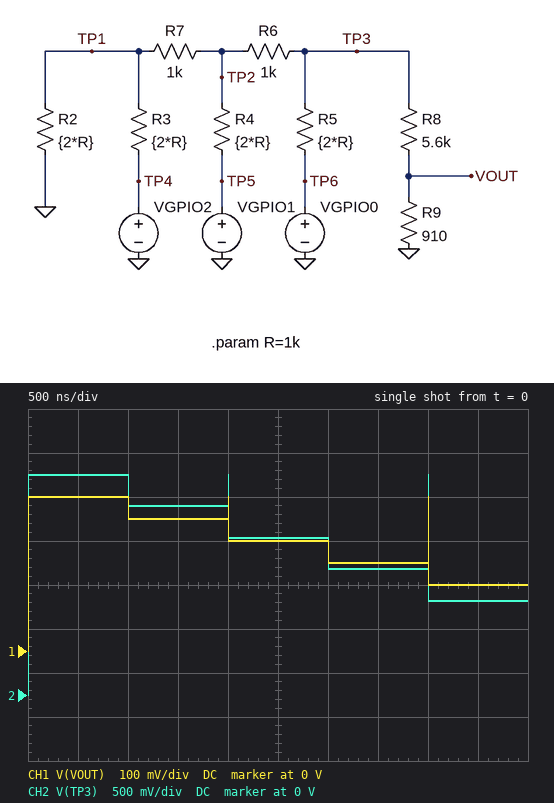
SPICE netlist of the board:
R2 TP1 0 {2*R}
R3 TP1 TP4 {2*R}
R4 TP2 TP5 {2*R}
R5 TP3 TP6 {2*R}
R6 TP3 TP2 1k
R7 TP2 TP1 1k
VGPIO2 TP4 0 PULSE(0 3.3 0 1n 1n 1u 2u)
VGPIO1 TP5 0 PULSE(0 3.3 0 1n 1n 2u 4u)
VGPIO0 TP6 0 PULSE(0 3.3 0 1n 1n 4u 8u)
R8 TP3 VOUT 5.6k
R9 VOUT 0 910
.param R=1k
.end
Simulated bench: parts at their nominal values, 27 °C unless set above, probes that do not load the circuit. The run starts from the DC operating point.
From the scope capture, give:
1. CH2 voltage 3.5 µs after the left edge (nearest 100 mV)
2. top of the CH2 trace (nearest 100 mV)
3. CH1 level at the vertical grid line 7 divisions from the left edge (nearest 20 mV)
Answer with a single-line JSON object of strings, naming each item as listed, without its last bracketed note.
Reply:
{"CH2 voltage 3.5 µs after the left edge": "1.4 V", "top of the CH2 trace": "2.5 V", "CH1 level at the vertical grid line 7 divisions from the left edge": "200 mV"}
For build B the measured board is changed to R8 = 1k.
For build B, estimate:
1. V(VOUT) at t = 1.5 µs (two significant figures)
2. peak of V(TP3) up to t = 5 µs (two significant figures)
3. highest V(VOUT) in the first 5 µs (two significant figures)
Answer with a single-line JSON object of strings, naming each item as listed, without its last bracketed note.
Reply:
{"V(VOUT) at t = 1.5 µs": "770 mV", "peak of V(TP3) up to t = 5 µs": "1.9 V", "highest V(VOUT) in the first 5 µs": "900 mV"}
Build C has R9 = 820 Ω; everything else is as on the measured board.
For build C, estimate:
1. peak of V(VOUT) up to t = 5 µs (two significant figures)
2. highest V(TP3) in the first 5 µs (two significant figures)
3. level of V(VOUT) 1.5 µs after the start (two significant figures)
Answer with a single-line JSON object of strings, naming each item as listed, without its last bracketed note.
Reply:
{"peak of V(VOUT) up to t = 5 µs": "320 mV", "highest V(TP3) in the first 5 µs": "2.5 V", "level of V(VOUT) 1.5 µs after the start": "270 mV"}
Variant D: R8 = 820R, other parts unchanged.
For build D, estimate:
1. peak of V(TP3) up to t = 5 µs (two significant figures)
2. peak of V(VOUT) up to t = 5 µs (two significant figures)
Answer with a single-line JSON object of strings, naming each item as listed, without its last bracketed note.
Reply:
{"peak of V(TP3) up to t = 5 µs": "1.8 V", "peak of V(VOUT) up to t = 5 µs": "960 mV"}
